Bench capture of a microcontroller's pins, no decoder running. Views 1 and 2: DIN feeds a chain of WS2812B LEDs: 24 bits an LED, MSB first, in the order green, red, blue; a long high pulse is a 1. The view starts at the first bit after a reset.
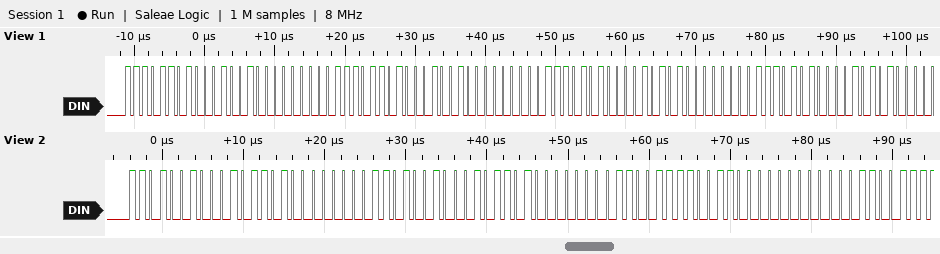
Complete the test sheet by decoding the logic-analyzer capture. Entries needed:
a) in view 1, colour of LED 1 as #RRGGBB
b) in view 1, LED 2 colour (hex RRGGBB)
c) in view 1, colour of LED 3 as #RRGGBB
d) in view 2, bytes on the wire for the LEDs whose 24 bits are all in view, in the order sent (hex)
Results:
#12ED00
#12ED00
#15EA00
D2 2D 00 D2 2D 00 CF 30 00
